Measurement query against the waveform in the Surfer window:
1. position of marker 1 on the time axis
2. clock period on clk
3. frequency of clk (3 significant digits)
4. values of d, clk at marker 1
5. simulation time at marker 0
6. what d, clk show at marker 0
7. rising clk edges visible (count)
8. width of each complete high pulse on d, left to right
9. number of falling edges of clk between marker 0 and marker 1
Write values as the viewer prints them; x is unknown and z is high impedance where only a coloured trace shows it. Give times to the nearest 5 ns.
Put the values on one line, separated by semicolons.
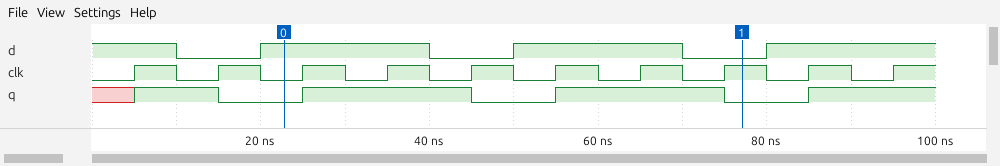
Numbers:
75 ns; 10 ns; 100 MHz; d=0, clk=1; 25 ns; d=1, clk=0; 10; 20 ns, 20 ns; 5
